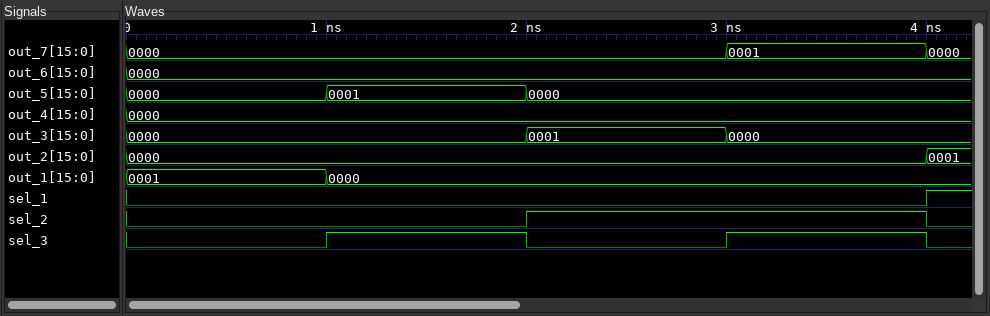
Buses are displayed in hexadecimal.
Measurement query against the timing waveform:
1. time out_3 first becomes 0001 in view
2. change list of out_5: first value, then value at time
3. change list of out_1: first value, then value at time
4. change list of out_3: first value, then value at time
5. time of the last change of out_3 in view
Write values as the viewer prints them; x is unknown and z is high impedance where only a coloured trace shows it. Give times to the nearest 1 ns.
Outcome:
2 ns
0000, 0001 at 1 ns, 0000 at 2 ns
0001, 0000 at 1 ns
0000, 0001 at 2 ns, 0000 at 3 ns
3 ns
